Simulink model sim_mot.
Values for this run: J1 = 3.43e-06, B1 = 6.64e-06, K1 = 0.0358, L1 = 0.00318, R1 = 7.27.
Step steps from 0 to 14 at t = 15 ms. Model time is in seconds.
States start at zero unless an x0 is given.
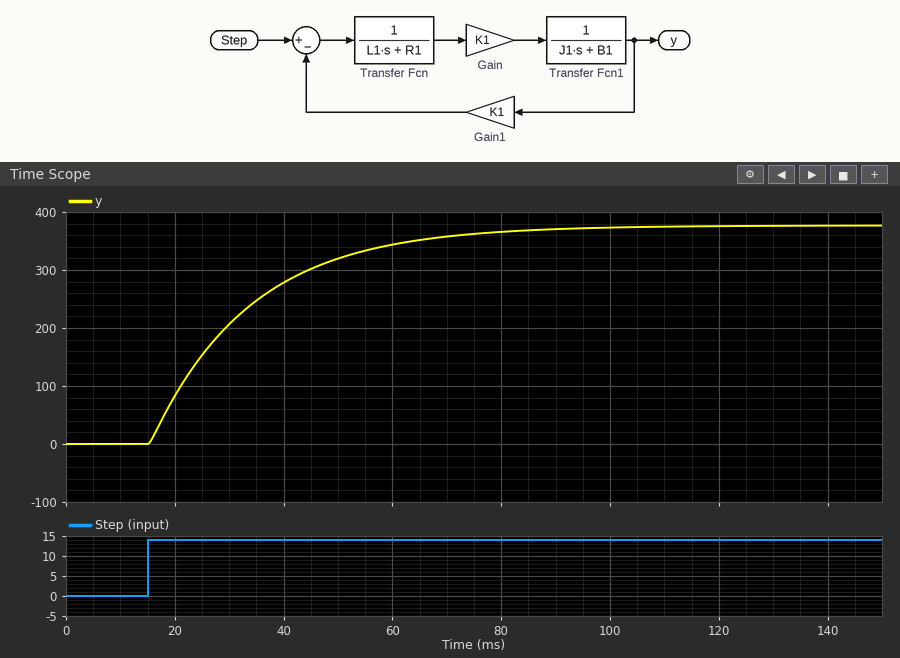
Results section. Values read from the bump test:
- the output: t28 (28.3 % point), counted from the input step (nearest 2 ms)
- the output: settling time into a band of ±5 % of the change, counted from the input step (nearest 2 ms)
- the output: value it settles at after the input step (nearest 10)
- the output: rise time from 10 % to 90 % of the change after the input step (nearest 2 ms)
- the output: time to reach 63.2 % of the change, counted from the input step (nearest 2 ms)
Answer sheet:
6 ms
56 ms
380
40 ms
18 ms
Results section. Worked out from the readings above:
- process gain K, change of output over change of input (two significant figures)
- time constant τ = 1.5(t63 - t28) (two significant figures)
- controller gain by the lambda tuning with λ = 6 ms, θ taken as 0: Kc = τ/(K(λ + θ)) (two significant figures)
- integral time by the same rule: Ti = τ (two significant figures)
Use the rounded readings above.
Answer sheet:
27
18 ms
0.11
18 ms
